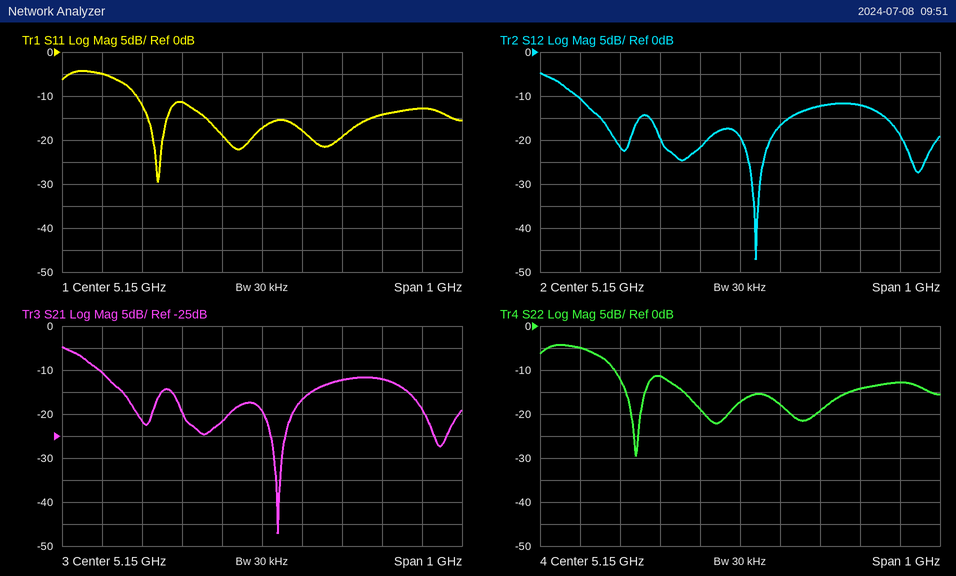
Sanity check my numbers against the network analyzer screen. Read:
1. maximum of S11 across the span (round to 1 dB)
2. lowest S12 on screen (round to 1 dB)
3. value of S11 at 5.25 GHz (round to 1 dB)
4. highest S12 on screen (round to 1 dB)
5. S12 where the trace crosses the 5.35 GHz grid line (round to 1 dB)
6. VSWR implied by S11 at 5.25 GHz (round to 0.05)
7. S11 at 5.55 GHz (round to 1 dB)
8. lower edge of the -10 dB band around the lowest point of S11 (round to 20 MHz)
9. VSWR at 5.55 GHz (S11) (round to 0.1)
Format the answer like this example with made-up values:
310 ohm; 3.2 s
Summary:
-4 dB; -47 dB; -18 dB; -5 dB; -12 dB; 1.30; -13 dB; 4.84 GHz; 1.6
